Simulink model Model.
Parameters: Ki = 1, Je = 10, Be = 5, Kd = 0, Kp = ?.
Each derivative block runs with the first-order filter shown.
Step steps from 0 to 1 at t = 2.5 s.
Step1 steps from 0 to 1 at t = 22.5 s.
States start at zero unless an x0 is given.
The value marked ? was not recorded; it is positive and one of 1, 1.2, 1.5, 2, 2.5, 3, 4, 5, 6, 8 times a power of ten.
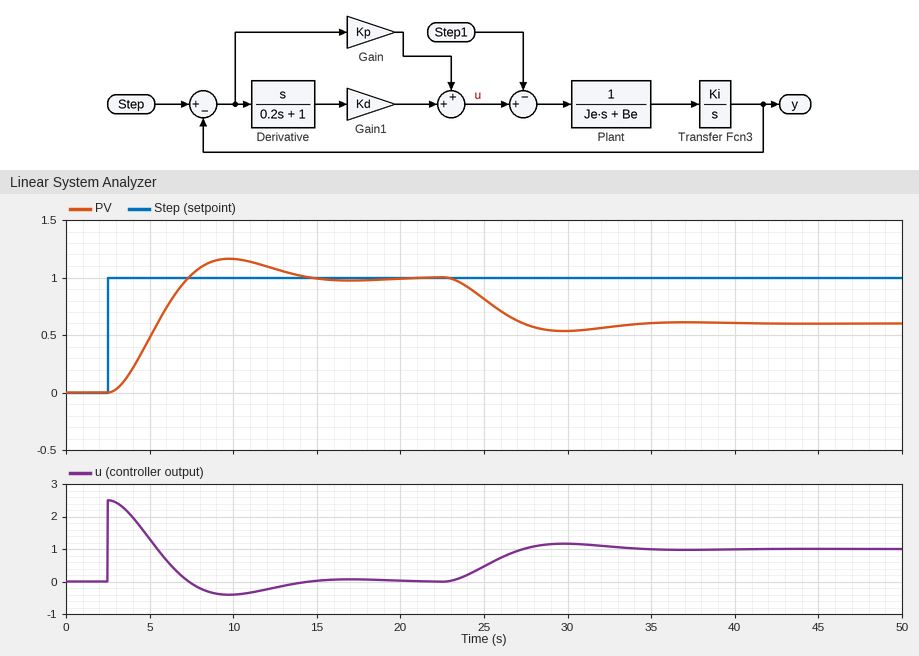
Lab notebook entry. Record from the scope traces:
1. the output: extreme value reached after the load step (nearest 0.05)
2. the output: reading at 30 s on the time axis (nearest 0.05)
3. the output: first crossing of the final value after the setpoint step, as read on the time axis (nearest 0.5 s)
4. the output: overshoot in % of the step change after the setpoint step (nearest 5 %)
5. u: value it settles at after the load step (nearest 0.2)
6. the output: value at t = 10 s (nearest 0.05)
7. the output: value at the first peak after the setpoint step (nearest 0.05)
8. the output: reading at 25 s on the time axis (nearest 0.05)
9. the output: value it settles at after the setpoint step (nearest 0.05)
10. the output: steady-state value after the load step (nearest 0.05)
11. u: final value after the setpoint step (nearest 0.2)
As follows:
0.55
0.55
7.5 s
15 %
1.0
1.15
1.15
0.80
1.00
0.60
0.0
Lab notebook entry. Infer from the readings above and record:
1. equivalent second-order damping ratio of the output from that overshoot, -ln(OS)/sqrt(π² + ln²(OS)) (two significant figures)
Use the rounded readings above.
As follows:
0.52
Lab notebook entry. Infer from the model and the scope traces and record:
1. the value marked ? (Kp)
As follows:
2.5
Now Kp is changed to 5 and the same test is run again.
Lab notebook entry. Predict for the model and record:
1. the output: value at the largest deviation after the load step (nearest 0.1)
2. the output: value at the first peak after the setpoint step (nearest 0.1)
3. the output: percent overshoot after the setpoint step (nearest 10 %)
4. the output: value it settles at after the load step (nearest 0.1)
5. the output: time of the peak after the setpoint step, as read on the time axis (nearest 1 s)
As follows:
0.7
1.3
30 %
0.8
7 s
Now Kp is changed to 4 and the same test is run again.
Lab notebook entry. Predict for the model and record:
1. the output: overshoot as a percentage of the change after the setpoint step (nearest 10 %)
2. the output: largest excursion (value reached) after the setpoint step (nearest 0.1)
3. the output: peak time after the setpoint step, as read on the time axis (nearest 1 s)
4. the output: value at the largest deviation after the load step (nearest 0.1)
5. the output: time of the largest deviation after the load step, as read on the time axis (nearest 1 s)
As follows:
30 %
1.3
8 s
0.7
28 s
